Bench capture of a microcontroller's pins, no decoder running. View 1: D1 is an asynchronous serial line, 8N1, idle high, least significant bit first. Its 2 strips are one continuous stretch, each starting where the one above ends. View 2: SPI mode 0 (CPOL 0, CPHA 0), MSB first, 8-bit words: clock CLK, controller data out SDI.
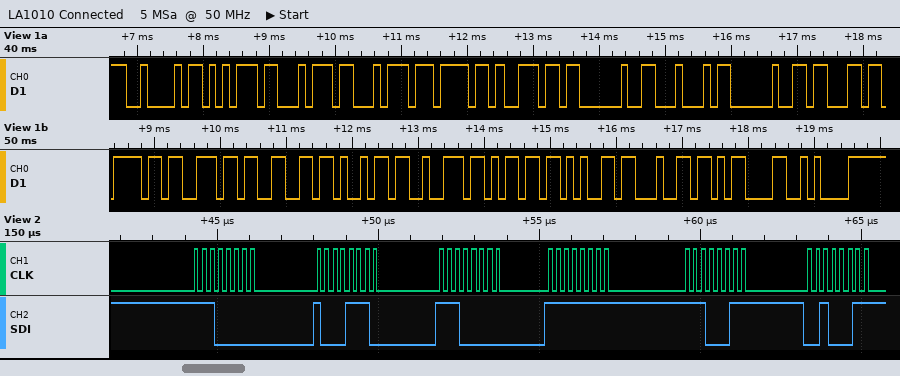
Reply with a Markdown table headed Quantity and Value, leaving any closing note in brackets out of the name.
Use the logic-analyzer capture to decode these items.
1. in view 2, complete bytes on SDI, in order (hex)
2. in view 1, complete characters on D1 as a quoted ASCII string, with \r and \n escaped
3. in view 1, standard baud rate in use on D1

| Quantity | Value |
|---|---|
| in view 2, complete bytes on SDI, in order | E0 8E E0 FF E3 23 |
| in view 1, complete characters on D1 as a quoted ASCII string, with \r and \n escaped | "Button D confirmed\r\n" |
| in view 1, standard baud rate in use on D1 | 9600 baud |
